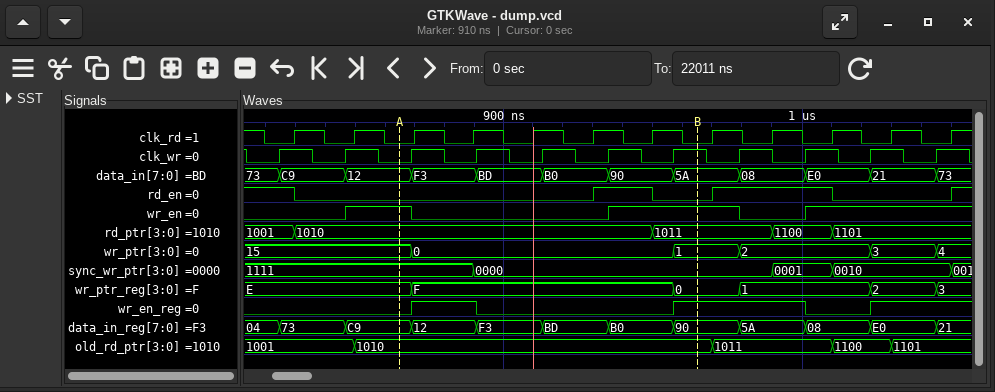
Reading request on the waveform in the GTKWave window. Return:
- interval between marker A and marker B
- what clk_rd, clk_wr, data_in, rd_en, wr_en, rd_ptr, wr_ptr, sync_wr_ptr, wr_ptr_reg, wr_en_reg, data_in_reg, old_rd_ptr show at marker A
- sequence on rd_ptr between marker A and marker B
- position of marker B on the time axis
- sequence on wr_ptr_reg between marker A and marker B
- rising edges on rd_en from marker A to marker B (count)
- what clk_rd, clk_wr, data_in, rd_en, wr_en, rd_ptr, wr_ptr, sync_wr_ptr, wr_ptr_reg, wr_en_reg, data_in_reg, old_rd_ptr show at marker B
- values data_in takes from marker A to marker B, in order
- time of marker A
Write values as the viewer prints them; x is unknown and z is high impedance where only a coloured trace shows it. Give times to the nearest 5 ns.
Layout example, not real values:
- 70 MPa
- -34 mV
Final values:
- 100 ns
- clk_rd=0, clk_wr=0, data_in=12, rd_en=0, wr_en=1, rd_ptr=1010, wr_ptr=15, sync_wr_ptr=1111, wr_ptr_reg=E, wr_en_reg=0, data_in_reg=C9, old_rd_ptr=1010
- 1010, 1011
- 965 ns
- E, F, 0
- 1
- clk_rd=0, clk_wr=1, data_in=5A, rd_en=0, wr_en=1, rd_ptr=1011, wr_ptr=1, sync_wr_ptr=0000, wr_ptr_reg=0, wr_en_reg=1, data_in_reg=90, old_rd_ptr=1010
- 12, F3, BD, B0, 90, 5A
- 865 ns
